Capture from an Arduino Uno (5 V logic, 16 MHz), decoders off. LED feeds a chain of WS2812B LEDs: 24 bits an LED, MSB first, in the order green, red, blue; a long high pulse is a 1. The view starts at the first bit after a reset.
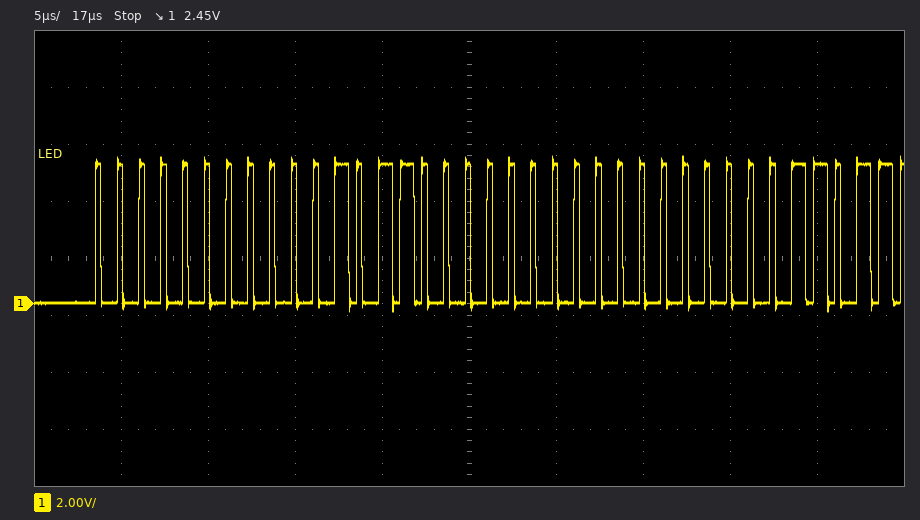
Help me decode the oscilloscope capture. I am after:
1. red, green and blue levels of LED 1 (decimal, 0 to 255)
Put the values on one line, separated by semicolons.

22, 0, 0
